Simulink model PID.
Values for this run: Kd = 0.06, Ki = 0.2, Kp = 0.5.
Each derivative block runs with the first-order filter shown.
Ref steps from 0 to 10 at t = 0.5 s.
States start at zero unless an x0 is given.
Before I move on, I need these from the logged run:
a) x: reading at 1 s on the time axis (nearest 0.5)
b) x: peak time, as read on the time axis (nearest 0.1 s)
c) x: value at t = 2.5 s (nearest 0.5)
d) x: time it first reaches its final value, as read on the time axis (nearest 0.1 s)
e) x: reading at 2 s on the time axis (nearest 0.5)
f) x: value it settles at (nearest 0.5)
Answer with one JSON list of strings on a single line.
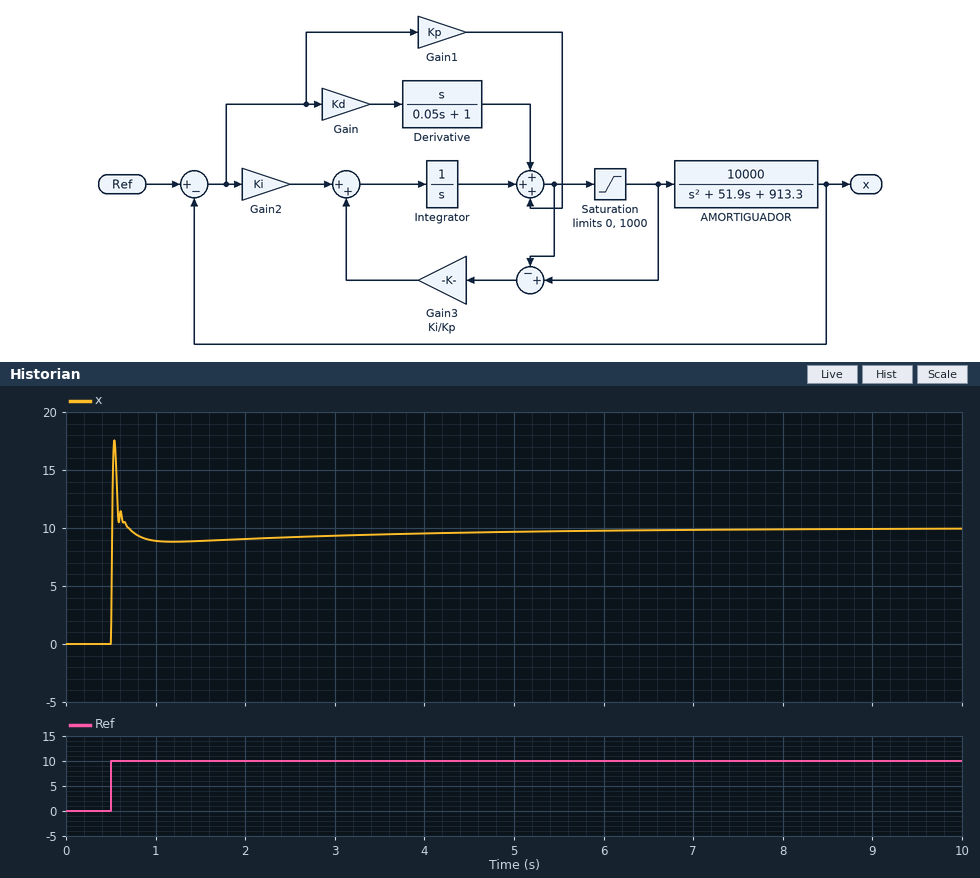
["9.0", "0.5 s", "9.0", "0.5 s", "9.0", "10.0"]
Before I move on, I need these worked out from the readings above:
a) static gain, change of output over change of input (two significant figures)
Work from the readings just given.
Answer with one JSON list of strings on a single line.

["1.0"]
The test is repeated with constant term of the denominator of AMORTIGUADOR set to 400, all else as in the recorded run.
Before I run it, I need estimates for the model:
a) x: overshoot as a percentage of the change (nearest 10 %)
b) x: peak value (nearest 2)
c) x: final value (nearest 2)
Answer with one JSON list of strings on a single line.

["100 %", "20", "10"]
